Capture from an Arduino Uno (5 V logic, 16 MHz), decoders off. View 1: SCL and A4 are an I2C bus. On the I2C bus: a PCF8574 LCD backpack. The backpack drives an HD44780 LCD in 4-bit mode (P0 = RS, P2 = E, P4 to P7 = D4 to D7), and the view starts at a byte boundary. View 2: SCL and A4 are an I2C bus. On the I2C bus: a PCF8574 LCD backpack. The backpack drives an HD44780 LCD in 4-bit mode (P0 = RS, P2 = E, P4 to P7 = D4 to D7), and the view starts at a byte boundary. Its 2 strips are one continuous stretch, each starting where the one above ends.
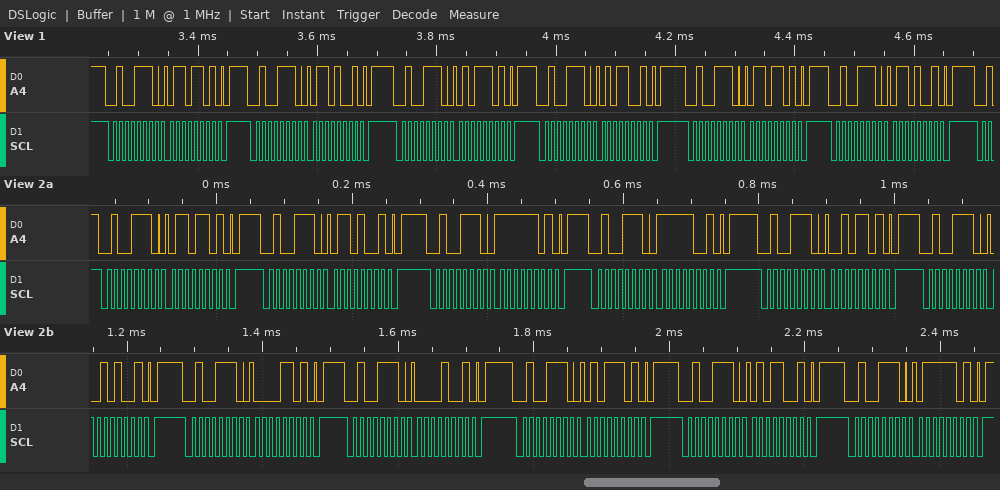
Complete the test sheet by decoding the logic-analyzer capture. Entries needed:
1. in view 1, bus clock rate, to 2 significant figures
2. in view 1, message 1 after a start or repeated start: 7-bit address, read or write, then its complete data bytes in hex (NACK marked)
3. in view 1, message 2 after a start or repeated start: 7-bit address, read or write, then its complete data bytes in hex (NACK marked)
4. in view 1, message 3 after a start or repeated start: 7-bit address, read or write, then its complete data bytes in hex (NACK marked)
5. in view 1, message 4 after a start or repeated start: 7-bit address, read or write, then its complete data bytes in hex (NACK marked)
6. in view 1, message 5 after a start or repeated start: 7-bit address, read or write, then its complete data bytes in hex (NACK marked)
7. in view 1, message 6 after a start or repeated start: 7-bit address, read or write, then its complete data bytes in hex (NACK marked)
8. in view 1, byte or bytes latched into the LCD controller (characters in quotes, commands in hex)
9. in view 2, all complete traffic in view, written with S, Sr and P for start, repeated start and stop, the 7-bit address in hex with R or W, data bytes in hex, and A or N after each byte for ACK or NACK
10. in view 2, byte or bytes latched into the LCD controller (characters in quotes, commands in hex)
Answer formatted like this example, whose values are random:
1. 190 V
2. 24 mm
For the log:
1. 100 kHz
2. 0x27 write: 6D
3. 0x27 write: 69
4. 0x27 write: 5D
5. 0x27 write: 59
6. 0x27 write: 6D
7. 0x27 write: 69
8. 'e'
9. S 27W A 6D A P S 27W A 69 A P S 27W A FD A P S 27W A F9 A P S 27W A 2D A P S 27W A 29 A P S 27W A 0D A P S 27W A 09 A P S 27W A 5D A P S 27W A 59 A P S 27W A 7D A P
10. 'o' ' '
